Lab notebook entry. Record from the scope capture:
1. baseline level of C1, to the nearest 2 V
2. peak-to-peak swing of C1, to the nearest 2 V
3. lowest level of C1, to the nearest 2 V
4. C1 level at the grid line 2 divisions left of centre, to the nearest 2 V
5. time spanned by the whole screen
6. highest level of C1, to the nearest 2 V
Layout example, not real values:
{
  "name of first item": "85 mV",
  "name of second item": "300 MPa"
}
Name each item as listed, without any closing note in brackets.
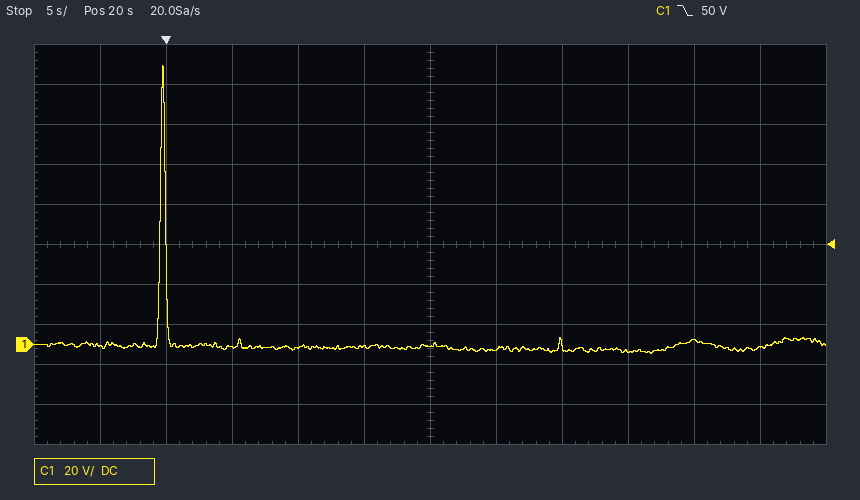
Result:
{
  "baseline level of C1, to the nearest 2 V": "-2 V",
  "peak-to-peak swing of C1, to the nearest 2 V": "144 V",
  "lowest level of C1, to the nearest 2 V": "-4 V",
  "C1 level at the grid line 2 divisions left of centre, to the nearest 2 V": "-2 V",
  "time spanned by the whole screen": "60 s",
  "highest level of C1, to the nearest 2 V": "140 V"
}
